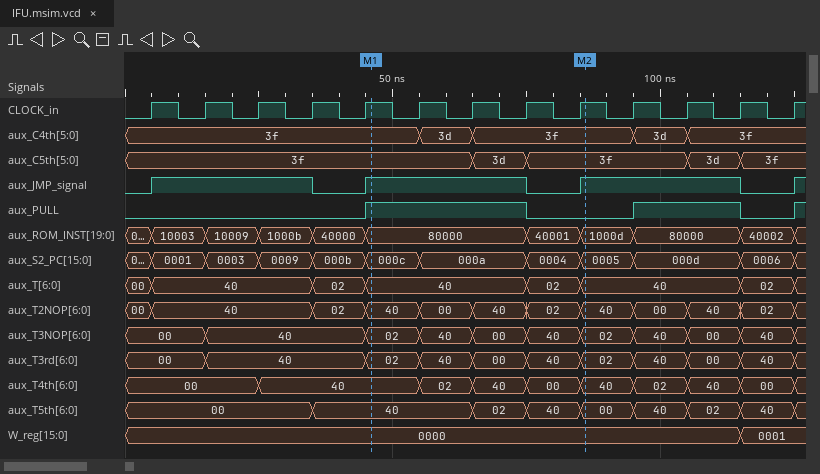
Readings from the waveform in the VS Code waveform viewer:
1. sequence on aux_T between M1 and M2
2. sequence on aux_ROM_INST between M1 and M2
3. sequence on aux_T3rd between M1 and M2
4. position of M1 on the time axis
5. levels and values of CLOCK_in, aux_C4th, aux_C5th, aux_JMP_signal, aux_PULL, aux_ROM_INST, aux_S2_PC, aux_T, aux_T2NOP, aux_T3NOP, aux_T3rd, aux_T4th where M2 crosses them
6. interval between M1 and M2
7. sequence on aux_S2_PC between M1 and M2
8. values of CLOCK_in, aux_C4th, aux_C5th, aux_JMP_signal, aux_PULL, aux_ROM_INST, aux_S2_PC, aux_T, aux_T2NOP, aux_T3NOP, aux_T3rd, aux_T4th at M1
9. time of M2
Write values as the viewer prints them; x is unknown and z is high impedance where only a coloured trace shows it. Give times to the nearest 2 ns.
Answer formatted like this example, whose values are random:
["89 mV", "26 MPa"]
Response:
["40, 02, 40", "80000, 40001, 1000d", "02, 40, 00, 40, 02", "46 ns", "CLOCK_in=1, aux_C4th=3f, aux_C5th=3f, aux_JMP_signal=1, aux_PULL=0, aux_ROM_INST=1000d, aux_S2_PC=0005, aux_T=40, aux_T2NOP=40, aux_T3NOP=02, aux_T3rd=02, aux_T4th=40", "40 ns", "000c, 000a, 0004, 0005", "CLOCK_in=1, aux_C4th=3f, aux_C5th=3f, aux_JMP_signal=1, aux_PULL=1, aux_ROM_INST=80000, aux_S2_PC=000c, aux_T=40, aux_T2NOP=40, aux_T3NOP=02, aux_T3rd=02, aux_T4th=40", "86 ns"]
